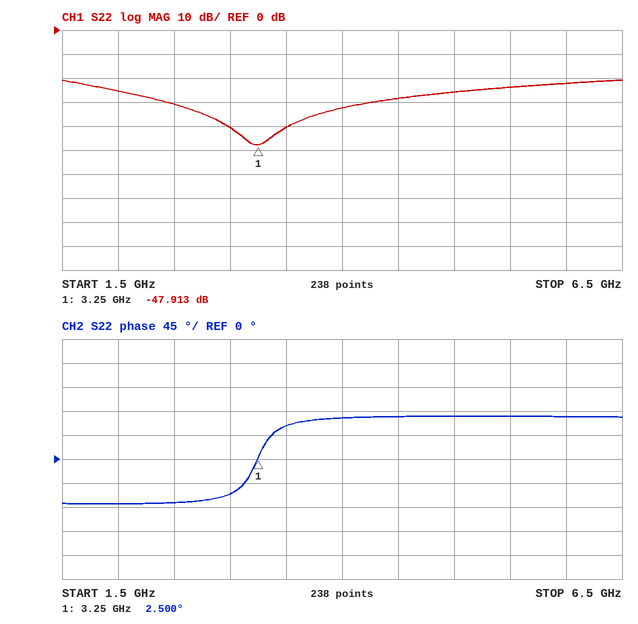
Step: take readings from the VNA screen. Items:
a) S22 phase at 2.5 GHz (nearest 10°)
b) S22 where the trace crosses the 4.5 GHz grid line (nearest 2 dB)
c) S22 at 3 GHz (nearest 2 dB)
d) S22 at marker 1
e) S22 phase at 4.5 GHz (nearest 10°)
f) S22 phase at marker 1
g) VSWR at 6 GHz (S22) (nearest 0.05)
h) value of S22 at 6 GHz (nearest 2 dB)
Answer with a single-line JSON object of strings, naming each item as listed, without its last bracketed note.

{"S22 phase at 2.5 GHz": "-80°", "S22 where the trace crosses the 4.5 GHz grid line": "-28 dB", "S22 at 3 GHz": "-40 dB", "S22 at marker 1": "-47.913 dB", "S22 phase at 4.5 GHz": "80°", "S22 phase at marker 1": "2.500°", "VSWR at 6 GHz (S22)": "1.15", "value of S22 at 6 GHz": "-22 dB"}
